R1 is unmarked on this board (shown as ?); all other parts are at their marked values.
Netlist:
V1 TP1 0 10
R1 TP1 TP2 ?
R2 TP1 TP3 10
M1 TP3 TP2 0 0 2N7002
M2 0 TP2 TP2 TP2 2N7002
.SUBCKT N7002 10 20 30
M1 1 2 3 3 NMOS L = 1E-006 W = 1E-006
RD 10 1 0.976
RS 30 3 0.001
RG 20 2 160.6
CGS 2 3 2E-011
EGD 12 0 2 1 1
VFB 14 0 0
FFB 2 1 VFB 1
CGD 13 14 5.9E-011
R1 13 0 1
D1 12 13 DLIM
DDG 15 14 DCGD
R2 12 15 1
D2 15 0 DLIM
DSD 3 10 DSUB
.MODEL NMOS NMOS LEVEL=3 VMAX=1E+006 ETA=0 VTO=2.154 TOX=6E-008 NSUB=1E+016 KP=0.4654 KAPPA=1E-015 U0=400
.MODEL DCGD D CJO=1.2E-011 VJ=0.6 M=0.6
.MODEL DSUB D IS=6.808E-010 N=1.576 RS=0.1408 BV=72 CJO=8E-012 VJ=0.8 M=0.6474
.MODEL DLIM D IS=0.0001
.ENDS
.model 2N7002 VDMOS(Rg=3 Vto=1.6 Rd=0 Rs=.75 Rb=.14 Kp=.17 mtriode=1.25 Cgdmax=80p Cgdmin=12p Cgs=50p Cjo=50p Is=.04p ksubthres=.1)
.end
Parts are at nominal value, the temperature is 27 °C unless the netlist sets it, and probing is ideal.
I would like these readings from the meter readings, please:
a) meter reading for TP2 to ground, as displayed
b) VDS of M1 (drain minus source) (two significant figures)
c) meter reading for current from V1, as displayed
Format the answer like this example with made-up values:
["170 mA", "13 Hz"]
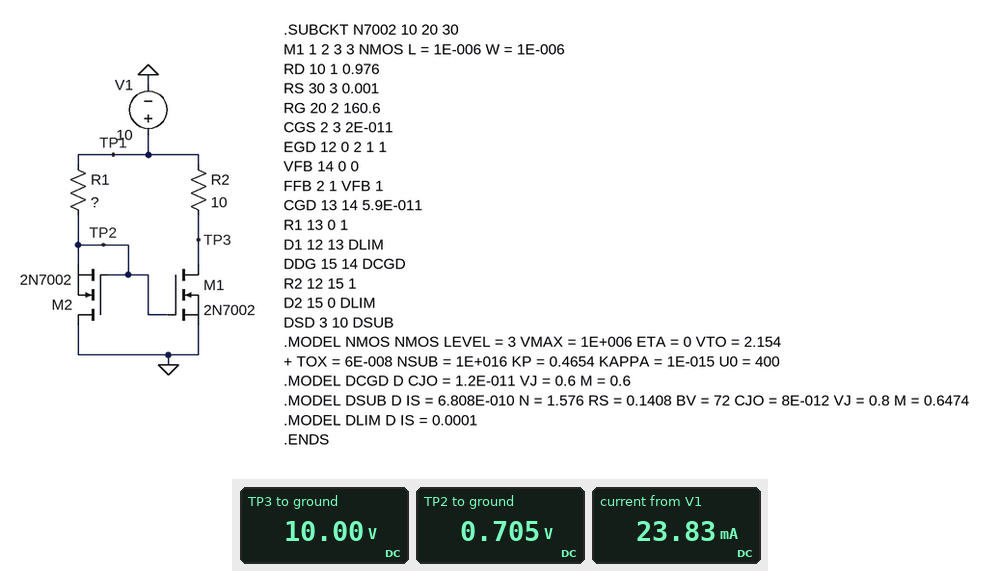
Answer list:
["0.705 V", "10 V", "23.83 mA"]
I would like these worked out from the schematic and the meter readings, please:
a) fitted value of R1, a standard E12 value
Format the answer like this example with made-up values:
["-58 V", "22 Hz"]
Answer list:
["390 Ω"]
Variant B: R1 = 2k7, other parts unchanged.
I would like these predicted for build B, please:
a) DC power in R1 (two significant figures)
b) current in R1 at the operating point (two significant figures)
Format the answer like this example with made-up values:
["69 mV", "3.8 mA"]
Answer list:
["32 mW", "3.5 mA"]
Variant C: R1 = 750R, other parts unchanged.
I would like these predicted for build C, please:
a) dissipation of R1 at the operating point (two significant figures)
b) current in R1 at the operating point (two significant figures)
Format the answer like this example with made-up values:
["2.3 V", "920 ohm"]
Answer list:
["120 mW", "12 mA"]
